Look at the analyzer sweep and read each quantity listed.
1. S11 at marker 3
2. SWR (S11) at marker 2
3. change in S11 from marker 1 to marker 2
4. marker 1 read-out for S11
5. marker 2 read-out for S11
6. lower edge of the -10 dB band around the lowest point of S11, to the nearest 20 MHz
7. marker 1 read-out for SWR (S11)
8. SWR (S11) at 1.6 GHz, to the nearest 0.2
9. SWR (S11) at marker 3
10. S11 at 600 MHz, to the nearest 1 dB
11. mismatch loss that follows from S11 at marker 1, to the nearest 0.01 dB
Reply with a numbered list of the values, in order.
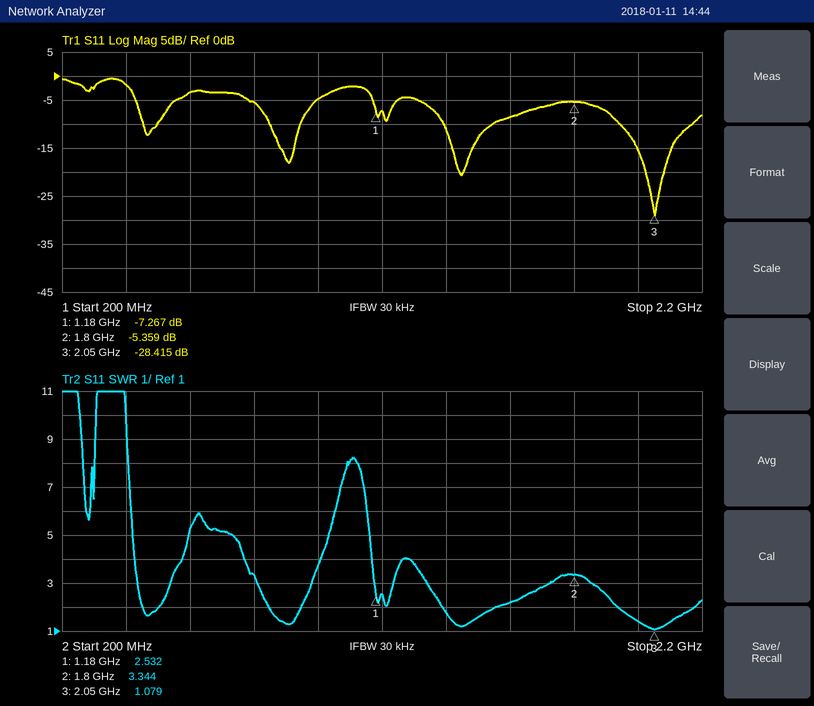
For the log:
1. -28.415 dB
2. 3.344
3. 1.908 dB
4. -7.267 dB
5. -5.359 dB
6. 1.94 GHz
7. 2.532
8. 2.2
9. 1.079
10. -3 dB
11. 0.90 dB
